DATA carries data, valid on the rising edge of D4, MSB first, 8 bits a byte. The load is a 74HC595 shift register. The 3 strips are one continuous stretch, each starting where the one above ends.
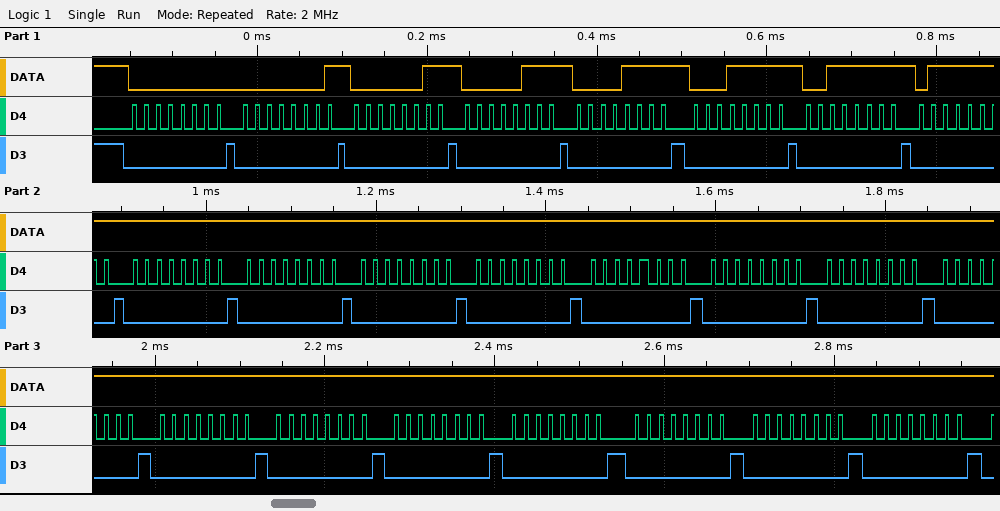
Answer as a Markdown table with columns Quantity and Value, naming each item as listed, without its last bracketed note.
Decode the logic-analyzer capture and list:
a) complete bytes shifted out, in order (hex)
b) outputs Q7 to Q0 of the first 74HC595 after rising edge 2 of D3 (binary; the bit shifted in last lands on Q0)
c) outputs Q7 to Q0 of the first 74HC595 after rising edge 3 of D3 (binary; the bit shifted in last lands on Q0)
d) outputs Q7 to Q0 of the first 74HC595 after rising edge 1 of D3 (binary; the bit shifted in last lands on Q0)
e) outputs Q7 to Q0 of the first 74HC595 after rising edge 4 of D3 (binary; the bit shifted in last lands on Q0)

| Quantity | Value |
|---|---|
| complete bytes shifted out, in order | 0x00 0x01 0x03 0x07 0x0F 0x1F 0x3F 0x7F 0xFF 0xFF 0xFF 0xFF 0xFF 0xFF 0xFF 0xFF 0xFF 0xFF 0xFF 0xFF 0xFF 0xFF 0xFF |
| outputs Q7 to Q0 of the first 74HC595 after rising edge 2 of D3 | 00000001 |
| outputs Q7 to Q0 of the first 74HC595 after rising edge 3 of D3 | 00000011 |
| outputs Q7 to Q0 of the first 74HC595 after rising edge 1 of D3 | 00000000 |
| outputs Q7 to Q0 of the first 74HC595 after rising edge 4 of D3 | 00000111 |
